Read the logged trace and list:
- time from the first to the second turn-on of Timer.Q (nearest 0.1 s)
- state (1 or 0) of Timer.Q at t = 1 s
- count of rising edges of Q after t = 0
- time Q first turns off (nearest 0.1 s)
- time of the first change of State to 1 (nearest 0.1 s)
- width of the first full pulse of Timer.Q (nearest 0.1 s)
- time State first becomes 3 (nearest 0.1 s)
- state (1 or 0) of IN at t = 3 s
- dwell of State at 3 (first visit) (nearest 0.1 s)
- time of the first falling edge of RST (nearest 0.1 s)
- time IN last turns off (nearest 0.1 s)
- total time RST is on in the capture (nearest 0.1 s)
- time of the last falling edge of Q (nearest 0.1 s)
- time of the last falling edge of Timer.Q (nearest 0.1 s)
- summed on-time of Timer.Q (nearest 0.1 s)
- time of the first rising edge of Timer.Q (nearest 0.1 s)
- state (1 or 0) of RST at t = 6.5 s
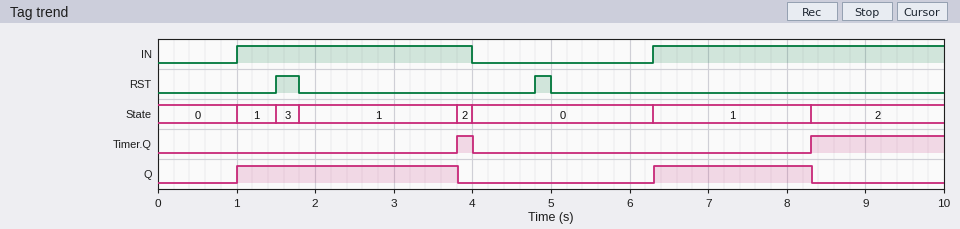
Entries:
4.5 s
0
2
3.8 s
1.0 s
0.2 s
1.5 s
1
0.3 s
1.8 s
4.0 s
0.5 s
8.3 s
4.0 s
1.9 s
3.8 s
0
